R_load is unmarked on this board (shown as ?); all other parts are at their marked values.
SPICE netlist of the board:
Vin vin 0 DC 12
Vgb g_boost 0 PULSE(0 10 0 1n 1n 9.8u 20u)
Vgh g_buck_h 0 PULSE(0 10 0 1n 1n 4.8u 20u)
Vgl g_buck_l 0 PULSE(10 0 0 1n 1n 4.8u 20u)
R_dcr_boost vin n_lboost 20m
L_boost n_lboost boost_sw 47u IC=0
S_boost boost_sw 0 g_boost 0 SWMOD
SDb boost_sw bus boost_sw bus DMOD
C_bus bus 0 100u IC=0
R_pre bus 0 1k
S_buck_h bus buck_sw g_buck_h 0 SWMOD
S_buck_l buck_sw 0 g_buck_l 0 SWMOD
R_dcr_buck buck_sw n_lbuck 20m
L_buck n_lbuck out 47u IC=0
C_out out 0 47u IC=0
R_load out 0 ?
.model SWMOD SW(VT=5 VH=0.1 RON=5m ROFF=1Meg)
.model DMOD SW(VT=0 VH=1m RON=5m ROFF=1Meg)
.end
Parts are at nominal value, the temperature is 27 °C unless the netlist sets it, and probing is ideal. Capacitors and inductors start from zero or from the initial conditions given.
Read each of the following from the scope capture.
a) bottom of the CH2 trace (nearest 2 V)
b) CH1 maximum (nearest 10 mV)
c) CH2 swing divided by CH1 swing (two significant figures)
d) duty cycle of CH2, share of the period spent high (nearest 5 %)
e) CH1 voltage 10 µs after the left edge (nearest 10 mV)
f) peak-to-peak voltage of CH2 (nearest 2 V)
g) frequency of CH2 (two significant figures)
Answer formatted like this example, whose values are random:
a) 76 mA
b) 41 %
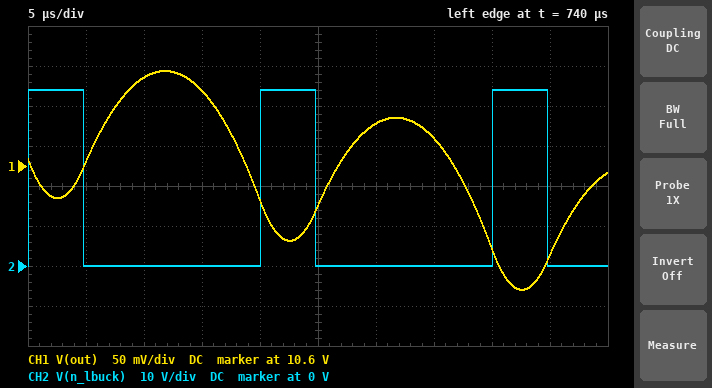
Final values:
a) 0 V
b) 10.72 V
c) 160
d) 25 %
e) 10.71 V
f) 44 V
g) 50 kHz
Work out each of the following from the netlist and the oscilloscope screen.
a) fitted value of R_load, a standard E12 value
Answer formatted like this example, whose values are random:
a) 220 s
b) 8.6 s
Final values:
a) 12 Ω
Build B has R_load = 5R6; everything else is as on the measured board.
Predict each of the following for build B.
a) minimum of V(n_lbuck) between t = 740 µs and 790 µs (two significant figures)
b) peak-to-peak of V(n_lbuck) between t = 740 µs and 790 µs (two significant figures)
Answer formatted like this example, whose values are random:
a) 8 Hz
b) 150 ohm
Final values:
a) -86 mV
b) 43 V
